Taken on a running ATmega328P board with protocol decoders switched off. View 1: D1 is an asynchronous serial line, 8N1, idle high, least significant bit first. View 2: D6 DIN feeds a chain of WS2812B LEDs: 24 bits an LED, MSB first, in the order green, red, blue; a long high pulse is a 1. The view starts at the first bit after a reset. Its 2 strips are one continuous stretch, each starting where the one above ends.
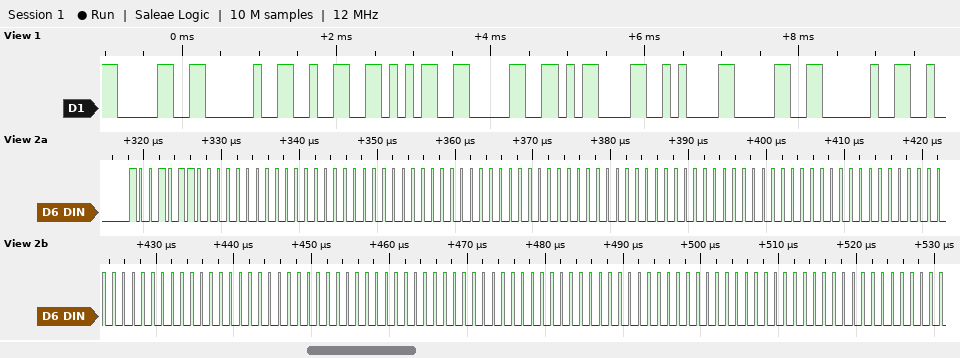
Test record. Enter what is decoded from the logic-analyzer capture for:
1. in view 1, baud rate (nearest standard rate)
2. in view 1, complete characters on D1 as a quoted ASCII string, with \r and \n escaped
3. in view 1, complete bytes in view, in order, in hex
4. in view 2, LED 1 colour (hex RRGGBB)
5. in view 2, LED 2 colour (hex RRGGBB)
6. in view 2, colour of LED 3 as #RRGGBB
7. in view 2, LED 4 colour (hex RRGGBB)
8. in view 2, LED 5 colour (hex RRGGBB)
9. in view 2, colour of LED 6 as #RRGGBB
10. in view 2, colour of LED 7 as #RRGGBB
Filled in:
9600 baud
"0 250\r\n0 "
30 20 32 35 30 0D 0A 30 20
#009600
#000000
#000000
#000000
#000000
#000000
#000000
